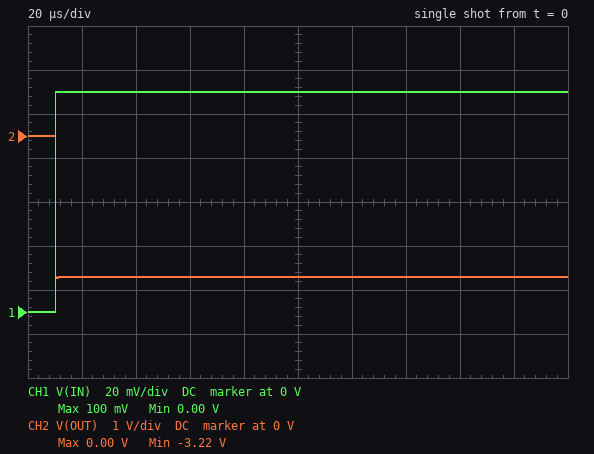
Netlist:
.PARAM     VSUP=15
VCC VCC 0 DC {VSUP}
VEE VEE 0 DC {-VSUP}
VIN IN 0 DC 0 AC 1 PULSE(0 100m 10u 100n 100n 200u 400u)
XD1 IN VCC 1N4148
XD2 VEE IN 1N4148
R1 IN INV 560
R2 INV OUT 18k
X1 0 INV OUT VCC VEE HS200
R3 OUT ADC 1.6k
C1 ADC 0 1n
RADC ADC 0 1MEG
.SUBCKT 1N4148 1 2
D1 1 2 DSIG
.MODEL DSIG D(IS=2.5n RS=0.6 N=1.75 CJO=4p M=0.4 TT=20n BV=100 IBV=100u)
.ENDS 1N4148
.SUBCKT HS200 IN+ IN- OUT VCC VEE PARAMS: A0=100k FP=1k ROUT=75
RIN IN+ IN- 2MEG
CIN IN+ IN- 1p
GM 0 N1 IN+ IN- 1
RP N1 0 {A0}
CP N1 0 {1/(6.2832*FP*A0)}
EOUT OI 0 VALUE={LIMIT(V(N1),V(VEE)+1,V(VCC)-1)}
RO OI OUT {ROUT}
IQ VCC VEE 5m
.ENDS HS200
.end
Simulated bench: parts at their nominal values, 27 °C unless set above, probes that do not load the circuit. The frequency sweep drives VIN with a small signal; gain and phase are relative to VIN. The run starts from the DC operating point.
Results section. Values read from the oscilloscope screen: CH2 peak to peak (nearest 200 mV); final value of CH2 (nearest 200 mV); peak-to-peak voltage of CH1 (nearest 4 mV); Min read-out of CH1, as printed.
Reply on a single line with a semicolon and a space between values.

3.2 V; -3.2 V; 100 mV; 0.00 V
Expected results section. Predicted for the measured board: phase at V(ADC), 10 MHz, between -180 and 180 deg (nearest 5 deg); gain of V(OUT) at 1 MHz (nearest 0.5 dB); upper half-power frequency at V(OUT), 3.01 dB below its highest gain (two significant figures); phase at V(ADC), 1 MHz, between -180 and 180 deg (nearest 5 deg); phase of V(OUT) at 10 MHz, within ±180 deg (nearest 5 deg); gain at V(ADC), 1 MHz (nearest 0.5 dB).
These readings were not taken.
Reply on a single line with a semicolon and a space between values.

15 deg; 29.5 dB; 2.9 MHz; 75 deg; 105 deg; 9.5 dB
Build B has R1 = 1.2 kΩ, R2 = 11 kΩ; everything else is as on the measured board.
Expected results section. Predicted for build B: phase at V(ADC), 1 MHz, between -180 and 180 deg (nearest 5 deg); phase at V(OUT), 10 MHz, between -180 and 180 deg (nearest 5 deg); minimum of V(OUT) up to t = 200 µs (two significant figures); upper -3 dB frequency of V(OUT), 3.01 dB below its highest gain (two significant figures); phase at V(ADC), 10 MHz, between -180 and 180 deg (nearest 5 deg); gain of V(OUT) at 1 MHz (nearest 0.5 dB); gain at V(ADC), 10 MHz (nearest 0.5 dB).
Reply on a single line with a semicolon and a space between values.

90 deg; 130 deg; -920 mV; 10 MHz; 40 deg; 19.0 dB; -24.0 dB
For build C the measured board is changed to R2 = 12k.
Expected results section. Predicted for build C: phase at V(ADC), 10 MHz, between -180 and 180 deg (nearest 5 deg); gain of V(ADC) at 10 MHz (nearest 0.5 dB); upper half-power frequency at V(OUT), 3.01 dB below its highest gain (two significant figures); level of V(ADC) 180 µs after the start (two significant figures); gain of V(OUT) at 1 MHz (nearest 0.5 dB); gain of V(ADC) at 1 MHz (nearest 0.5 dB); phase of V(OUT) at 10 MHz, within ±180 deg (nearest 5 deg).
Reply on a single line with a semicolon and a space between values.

20 deg; -21.5 dB; 4.3 MHz; -2.1 V; 26.5 dB; 6.5 dB; 110 deg
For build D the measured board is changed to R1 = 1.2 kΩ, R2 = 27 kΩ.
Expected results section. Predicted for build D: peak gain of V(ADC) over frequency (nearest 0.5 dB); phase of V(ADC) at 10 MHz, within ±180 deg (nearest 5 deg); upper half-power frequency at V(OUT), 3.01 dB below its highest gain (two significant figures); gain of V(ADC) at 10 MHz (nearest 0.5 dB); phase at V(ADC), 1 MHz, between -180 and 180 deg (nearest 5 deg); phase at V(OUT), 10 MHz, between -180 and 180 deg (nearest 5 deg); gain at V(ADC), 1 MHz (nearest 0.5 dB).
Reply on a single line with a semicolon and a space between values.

27.0 dB; 20 deg; 4.2 MHz; -21.5 dB; 80 deg; 110 deg; 6.5 dB
